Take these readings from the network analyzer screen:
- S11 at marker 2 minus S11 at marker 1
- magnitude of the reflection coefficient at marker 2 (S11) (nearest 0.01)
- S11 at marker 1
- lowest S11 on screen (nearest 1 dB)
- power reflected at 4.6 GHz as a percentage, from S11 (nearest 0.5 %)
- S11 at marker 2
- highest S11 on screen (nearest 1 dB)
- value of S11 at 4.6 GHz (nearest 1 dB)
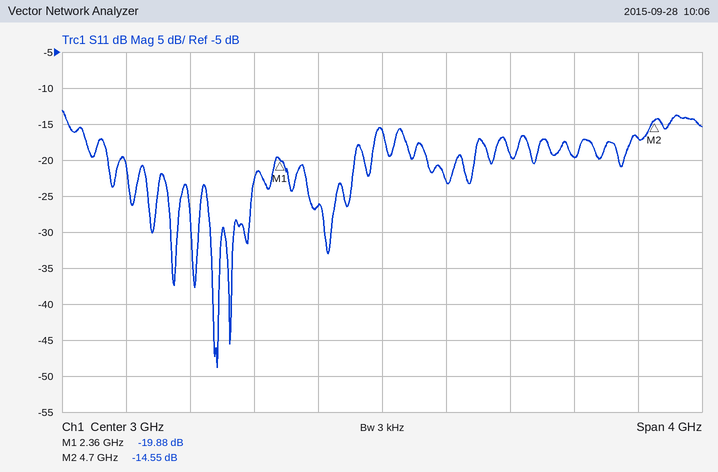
5.33 dB
0.19
-19.88 dB
-49 dB
2.0 %
-14.55 dB
-13 dB
-17 dB
